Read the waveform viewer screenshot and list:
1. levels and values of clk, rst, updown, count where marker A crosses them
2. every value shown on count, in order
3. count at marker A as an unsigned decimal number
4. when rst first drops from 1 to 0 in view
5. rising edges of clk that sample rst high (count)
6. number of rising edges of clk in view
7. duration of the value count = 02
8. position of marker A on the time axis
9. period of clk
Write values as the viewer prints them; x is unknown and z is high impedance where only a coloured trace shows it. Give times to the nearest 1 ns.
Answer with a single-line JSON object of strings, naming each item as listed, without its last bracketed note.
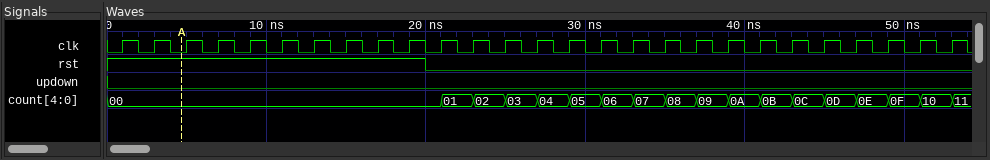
{"levels and values of clk, rst, updown, count where marker A crosses them": "clk=0, rst=1, updown=0, count=00", "every value shown on count, in order": "00, 01, 02, 03, 04, 05, 06, 07, 08, 09, 0A, 0B, 0C, 0D, 0E, 0F, 10, 11", "count at marker A as an unsigned decimal number": "0", "when rst first drops from 1 to 0 in view": "20 ns", "rising edges of clk that sample rst high": "10", "number of rising edges of clk in view": "27", "duration of the value count = 02": "2 ns", "position of marker A on the time axis": "5 ns", "period of clk": "2 ns"}
